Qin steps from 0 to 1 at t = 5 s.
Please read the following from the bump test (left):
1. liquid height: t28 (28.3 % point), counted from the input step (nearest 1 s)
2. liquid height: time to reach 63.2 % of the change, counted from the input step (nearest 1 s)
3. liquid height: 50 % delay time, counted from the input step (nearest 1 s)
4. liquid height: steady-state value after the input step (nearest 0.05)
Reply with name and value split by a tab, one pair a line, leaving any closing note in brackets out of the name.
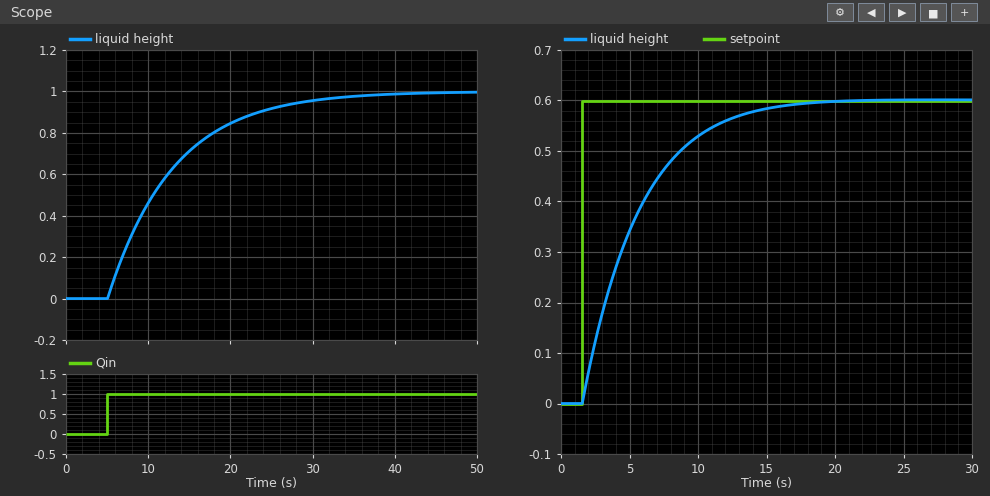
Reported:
liquid height: t28 (28.3 % point), counted from the input step	3 s
liquid height: time to reach 63.2 % of the change, counted from the input step	8 s
liquid height: 50 % delay time, counted from the input step	6 s
liquid height: steady-state value after the input step	1.00
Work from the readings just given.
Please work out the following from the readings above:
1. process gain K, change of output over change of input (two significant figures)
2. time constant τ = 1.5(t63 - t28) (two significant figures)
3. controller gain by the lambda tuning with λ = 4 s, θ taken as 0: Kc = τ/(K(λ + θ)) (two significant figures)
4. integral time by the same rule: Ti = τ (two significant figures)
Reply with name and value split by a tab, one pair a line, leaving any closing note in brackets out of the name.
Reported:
process gain K, change of output over change of input	1.0
time constant τ = 1.5(t63 - t28)	7.5 s
controller gain by the lambda tuning with λ = 4 s, θ taken as 0: Kc = τ/(K(λ + θ))	1.9
integral time by the same rule: Ti = τ	7.5 s
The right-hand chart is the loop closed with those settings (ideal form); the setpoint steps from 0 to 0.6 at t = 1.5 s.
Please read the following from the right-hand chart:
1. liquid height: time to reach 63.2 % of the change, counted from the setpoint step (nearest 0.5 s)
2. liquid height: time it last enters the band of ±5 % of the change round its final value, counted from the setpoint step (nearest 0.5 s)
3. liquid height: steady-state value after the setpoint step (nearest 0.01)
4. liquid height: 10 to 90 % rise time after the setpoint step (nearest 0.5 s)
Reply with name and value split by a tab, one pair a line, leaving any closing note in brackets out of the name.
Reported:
liquid height: time to reach 63.2 % of the change, counted from the setpoint step	4.0 s
liquid height: time it last enters the band of ±5 % of the change round its final value, counted from the setpoint step	11.5 s
liquid height: steady-state value after the setpoint step	0.60
liquid height: 10 to 90 % rise time after the setpoint step	8.5 s
